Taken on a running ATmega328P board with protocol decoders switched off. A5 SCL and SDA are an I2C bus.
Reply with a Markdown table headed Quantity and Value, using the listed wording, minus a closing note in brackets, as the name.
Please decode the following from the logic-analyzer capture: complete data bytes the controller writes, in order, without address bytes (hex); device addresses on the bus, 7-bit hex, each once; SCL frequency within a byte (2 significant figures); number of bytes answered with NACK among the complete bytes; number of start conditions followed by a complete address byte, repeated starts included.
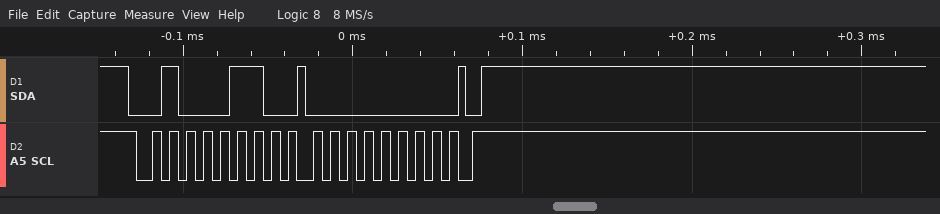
| Quantity | Value |
|---|---|
| complete data bytes the controller writes, in order, without address bytes | 00 |
| device addresses on the bus, 7-bit hex, each once | 0x23 |
| SCL frequency within a byte | 100 kHz |
| number of bytes answered with NACK among the complete bytes | 0 |
| number of start conditions followed by a complete address byte, repeated starts included | 1 |
